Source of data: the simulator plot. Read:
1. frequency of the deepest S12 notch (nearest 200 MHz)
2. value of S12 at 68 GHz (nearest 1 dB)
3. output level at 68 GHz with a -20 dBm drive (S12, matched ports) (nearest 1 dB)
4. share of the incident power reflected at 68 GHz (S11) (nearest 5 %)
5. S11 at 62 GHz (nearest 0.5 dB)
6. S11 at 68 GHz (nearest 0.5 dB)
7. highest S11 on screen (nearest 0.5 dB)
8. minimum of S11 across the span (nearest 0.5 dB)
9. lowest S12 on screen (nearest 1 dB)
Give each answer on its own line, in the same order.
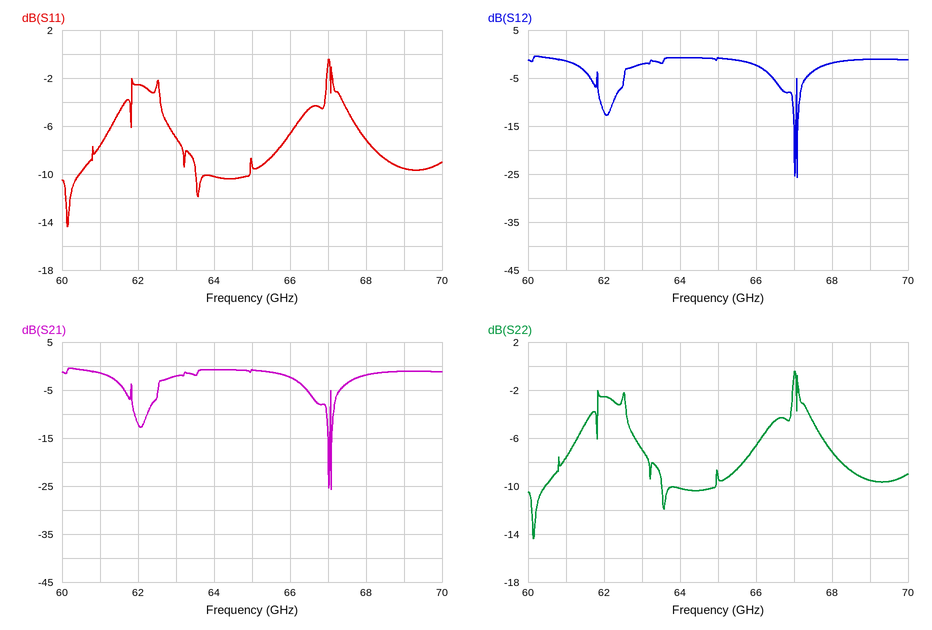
67.0 GHz
-2 dB
-22 dBm
20 %
-2.5 dB
-7.0 dB
-0.5 dB
-14.5 dB
-26 dB
